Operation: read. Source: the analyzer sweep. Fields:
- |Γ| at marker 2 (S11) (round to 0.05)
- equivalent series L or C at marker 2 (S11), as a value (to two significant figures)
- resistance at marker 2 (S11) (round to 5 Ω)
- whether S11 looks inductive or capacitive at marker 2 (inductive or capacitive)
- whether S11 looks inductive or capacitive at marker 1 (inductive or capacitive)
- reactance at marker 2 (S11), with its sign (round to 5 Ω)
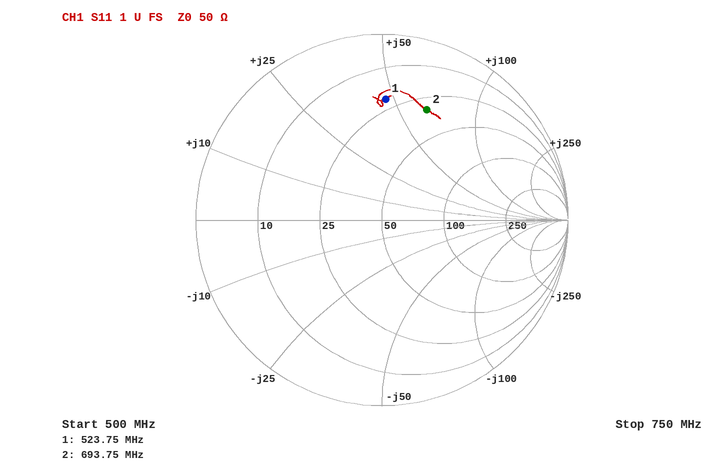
0.65
15 nH
30 Ω
inductive
inductive
+65 Ω
